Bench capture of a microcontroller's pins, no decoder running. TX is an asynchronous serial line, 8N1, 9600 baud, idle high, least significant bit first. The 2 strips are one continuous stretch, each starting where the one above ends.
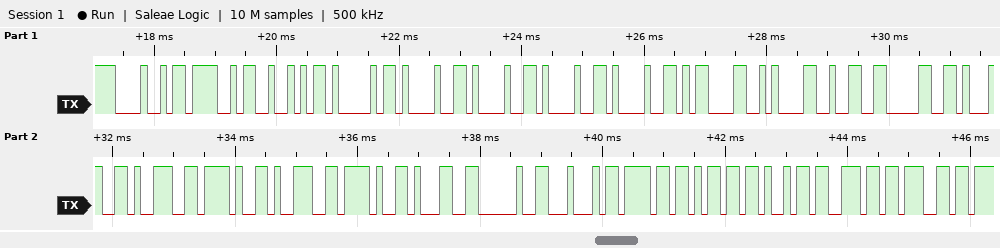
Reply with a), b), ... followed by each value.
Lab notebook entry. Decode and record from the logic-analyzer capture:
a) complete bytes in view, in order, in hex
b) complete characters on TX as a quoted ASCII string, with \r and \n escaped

a) 48 4F 52 41 21 21 21 21 0D 0A 32 30 31 39 2F 39 2F 31 20 44 6F 6D 69 6E 67
b) "HORA!!!!\r\n2019/9/1 Doming"
